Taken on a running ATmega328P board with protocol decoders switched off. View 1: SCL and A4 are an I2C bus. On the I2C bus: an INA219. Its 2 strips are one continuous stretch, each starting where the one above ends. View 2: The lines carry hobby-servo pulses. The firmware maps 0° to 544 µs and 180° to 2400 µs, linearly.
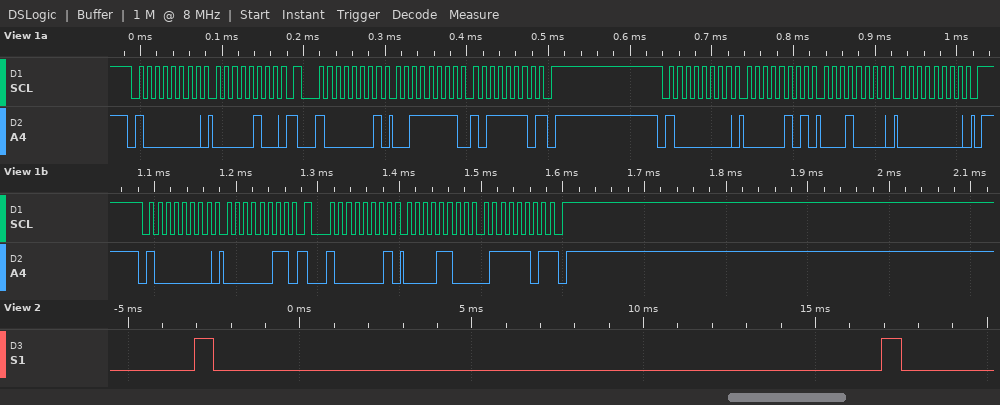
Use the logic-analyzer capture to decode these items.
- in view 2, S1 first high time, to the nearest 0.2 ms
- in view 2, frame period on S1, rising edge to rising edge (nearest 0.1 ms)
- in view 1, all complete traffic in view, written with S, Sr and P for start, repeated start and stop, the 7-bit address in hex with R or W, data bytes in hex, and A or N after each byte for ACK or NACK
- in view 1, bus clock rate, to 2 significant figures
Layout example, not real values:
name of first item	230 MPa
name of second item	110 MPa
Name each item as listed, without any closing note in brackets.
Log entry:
in view 2, S1 first high time, to the nearest 0.2 ms	0.6 ms
in view 2, frame period on S1, rising edge to rising edge	20.0 ms
in view 1, all complete traffic in view, written with S, Sr and P for start, repeated start and stop, the 7-bit address in hex with R or W, data bytes in hex, and A or N after each byte for ACK or NACK	S 40W A 04 A Sr 40R A 3F A BE N P S 40W A 05 A 10 A 00 A P S 40W A 03 A Sr 40R A 0C A 7D N P
in view 1, bus clock rate, to 2 significant figures	100 kHz
